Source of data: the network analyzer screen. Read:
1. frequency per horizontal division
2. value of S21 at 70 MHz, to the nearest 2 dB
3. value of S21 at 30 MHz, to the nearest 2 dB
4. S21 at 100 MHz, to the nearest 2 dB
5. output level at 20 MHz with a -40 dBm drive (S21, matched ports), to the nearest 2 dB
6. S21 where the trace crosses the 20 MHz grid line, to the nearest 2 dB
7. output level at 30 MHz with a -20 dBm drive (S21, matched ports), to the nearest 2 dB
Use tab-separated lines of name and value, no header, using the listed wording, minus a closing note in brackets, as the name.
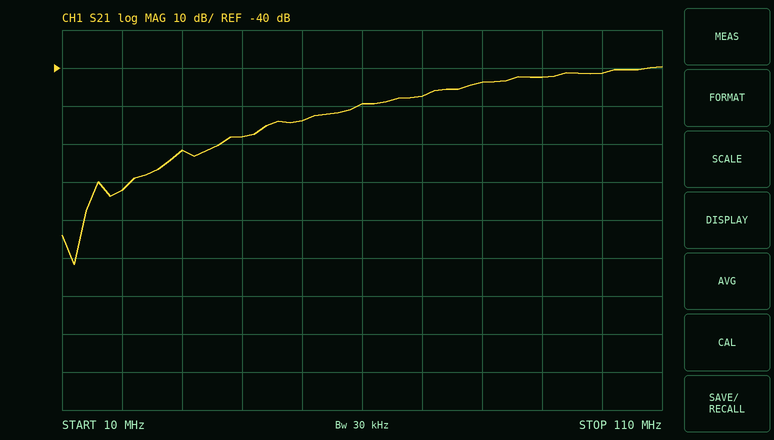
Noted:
frequency per horizontal division	10 MHz
value of S21 at 70 MHz, to the nearest 2 dB	-48 dB
value of S21 at 30 MHz, to the nearest 2 dB	-62 dB
S21 at 100 MHz, to the nearest 2 dB	-42 dB
output level at 20 MHz with a -40 dBm drive (S21, matched ports), to the nearest 2 dB	-112 dBm
S21 where the trace crosses the 20 MHz grid line, to the nearest 2 dB	-72 dB
output level at 30 MHz with a -20 dBm drive (S21, matched ports), to the nearest 2 dB	-82 dBm
